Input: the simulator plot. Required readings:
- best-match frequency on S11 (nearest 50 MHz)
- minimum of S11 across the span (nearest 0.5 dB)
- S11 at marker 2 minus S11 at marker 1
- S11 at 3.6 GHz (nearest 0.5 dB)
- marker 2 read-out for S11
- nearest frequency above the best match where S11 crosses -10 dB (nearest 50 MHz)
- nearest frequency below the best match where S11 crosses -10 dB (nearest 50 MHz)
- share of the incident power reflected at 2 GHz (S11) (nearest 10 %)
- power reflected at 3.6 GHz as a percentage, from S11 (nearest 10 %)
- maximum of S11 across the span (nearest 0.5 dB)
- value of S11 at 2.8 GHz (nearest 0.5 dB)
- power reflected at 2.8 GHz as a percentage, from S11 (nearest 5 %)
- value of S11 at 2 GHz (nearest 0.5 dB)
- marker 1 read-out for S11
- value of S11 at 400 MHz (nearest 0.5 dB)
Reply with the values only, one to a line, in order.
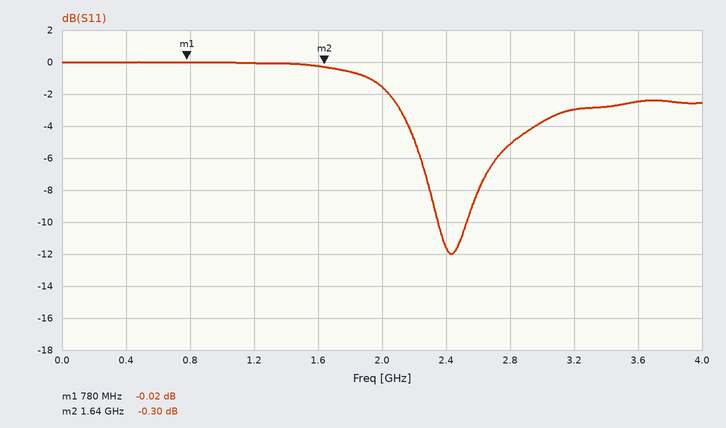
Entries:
2.45 GHz
-12.0 dB
-0.28 dB
-2.5 dB
-0.30 dB
2.55 GHz
2.35 GHz
70 %
60 %
0.0 dB
-5.0 dB
30 %
-1.5 dB
-0.02 dB
0.0 dB
